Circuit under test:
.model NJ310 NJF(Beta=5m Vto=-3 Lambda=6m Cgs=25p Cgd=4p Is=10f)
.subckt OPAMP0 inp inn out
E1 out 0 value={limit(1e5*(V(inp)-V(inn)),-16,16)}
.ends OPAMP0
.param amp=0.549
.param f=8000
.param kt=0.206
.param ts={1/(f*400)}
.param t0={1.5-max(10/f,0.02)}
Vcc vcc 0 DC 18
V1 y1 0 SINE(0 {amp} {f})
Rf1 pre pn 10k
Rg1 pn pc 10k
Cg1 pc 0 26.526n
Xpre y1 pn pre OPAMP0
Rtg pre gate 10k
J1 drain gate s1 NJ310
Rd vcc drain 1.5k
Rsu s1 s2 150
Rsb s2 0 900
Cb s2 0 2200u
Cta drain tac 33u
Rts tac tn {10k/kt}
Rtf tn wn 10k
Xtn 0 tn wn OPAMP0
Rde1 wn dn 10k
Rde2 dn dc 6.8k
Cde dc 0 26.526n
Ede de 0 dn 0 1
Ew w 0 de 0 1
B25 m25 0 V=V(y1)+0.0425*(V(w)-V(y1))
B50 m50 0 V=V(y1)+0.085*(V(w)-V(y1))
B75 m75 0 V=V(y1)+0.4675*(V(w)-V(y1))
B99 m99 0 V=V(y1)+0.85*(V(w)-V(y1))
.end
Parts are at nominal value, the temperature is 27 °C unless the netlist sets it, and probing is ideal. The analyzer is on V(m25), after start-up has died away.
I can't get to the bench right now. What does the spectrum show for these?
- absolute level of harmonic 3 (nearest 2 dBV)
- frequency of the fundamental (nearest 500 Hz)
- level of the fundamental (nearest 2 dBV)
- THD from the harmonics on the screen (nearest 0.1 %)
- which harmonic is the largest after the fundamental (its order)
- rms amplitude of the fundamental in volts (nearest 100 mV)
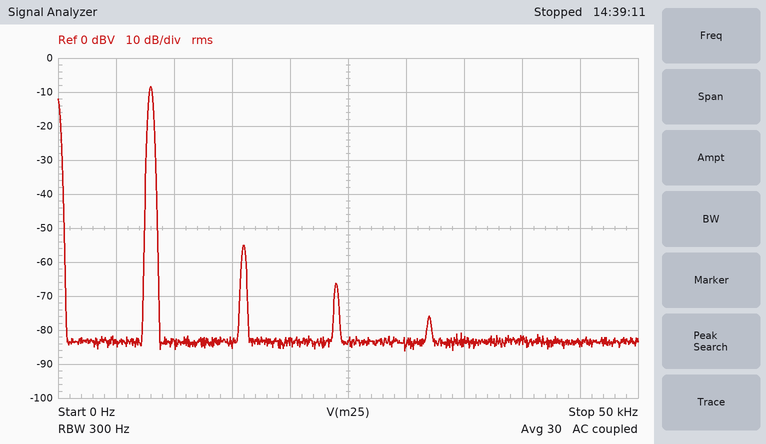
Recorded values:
-66 dBV
8.0 kHz
-8 dBV
0.5 %
2
400 mV
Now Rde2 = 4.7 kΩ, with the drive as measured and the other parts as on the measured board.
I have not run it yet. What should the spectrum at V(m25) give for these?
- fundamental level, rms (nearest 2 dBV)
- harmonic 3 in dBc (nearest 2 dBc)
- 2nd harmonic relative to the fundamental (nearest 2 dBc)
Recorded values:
-8 dBV
-60 dBc
-48 dBc
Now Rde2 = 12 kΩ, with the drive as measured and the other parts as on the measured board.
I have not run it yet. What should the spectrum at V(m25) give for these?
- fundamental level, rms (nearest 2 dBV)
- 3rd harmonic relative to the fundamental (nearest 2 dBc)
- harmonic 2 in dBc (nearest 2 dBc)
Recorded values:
-8 dBV
-56 dBc
-44 dBc
